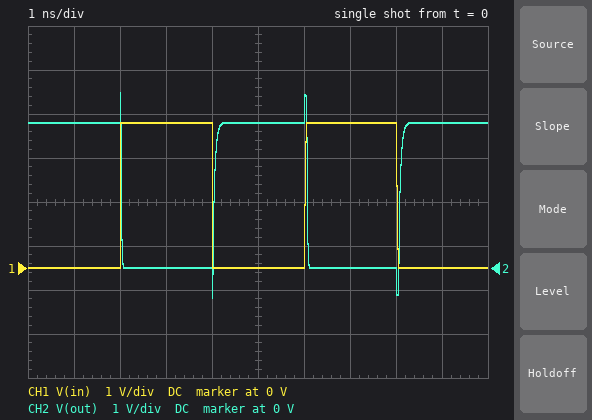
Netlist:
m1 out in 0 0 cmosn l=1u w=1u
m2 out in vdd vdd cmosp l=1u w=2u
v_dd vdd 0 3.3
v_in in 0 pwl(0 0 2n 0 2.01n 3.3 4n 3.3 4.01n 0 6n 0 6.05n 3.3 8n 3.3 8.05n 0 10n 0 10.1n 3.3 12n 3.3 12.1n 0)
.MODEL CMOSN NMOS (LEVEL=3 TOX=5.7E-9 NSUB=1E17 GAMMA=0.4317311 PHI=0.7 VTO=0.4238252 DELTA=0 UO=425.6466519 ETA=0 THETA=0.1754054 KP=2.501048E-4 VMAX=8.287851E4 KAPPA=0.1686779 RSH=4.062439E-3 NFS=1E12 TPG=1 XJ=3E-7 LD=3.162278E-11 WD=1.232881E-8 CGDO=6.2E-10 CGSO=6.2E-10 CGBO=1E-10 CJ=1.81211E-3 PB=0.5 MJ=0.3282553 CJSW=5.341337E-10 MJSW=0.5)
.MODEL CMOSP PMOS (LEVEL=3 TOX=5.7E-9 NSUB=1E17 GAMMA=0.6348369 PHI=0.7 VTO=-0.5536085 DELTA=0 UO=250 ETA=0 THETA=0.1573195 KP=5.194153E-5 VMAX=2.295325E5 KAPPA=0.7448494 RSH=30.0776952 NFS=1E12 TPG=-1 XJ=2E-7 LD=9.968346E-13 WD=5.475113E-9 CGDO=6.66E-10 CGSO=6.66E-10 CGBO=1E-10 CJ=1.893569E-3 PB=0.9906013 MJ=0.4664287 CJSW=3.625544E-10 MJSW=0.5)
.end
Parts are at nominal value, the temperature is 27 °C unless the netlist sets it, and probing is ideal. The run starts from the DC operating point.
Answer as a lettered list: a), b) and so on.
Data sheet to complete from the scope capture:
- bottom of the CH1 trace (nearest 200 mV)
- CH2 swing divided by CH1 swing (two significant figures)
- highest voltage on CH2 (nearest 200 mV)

a) 0 V
b) 1.4
c) 4.0 V
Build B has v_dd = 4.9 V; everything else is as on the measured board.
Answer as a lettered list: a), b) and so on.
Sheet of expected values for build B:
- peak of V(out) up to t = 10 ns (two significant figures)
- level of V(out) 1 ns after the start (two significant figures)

a) 5.6 V
b) 4.9 V
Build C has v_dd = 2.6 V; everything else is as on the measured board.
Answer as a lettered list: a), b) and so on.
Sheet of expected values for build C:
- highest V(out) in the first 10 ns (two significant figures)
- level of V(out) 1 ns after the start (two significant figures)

a) 3.3 V
b) 2.6 V
